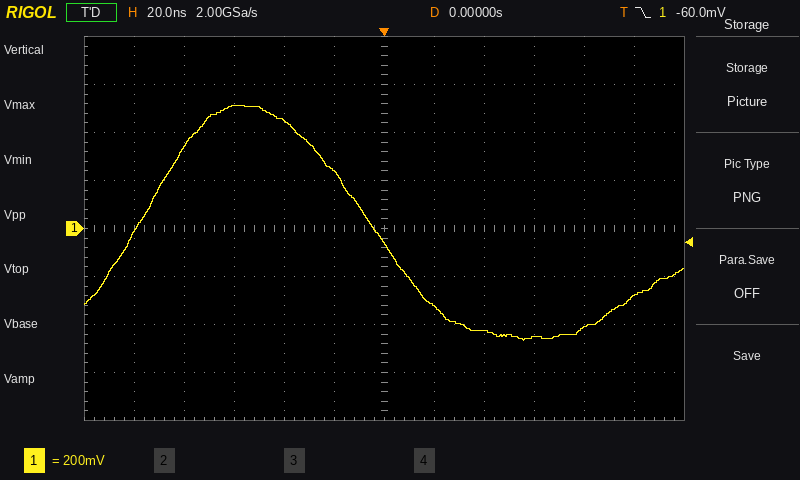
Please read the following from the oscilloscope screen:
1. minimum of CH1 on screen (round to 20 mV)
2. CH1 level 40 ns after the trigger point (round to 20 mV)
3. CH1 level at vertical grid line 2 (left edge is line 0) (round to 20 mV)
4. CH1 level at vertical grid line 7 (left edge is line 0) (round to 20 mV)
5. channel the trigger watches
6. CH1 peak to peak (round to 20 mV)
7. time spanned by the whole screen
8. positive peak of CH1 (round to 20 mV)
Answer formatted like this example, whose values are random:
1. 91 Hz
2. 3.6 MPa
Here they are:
1. -460 mV
2. -420 mV
3. 340 mV
4. -320 mV
5. CH1
6. 980 mV
7. 240 ns
8. 520 mV
